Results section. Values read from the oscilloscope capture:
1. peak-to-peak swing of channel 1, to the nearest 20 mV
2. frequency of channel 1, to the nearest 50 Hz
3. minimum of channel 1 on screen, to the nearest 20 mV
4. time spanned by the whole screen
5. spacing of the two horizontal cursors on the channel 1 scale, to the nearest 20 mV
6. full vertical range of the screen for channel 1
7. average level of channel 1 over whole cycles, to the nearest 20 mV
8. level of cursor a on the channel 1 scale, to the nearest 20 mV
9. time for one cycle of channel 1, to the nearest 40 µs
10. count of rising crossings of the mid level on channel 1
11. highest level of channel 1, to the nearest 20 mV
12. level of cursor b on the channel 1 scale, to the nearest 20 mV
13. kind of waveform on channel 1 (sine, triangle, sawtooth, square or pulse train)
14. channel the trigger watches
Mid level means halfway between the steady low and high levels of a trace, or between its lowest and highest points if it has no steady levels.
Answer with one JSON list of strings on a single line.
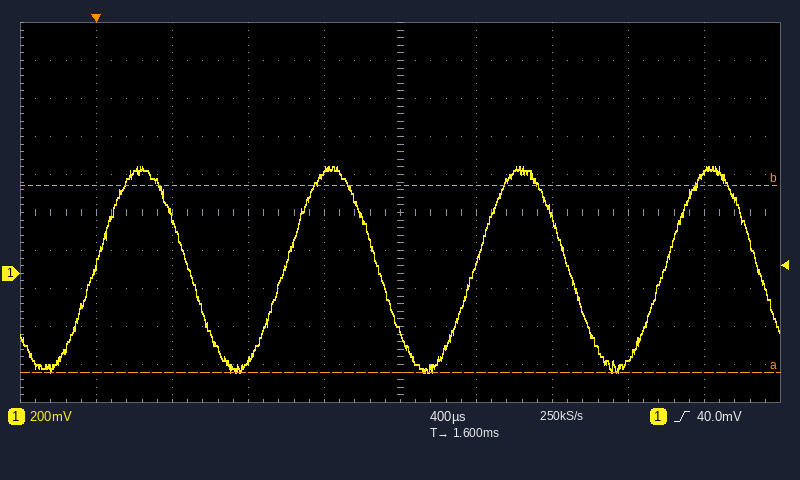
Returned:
["1.08 V", "1.00 kHz", "-520 mV", "4 ms", "980 mV", "2 V", "20 mV", "-520 mV", "1.00 ms", "4", "560 mV", "460 mV", "sine", "channel 1"]
